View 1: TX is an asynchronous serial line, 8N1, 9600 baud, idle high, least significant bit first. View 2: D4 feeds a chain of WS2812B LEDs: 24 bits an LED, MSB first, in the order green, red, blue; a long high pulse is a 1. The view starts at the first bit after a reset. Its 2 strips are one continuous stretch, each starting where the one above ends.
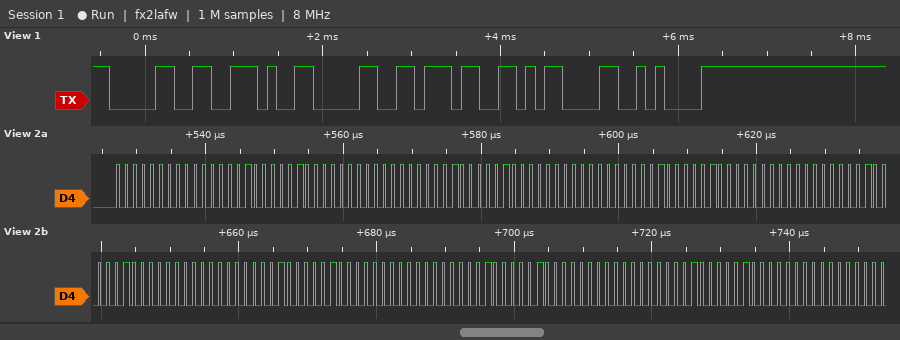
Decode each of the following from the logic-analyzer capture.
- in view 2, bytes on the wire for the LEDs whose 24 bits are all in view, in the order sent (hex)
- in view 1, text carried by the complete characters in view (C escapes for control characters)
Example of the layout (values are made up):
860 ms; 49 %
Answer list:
00 01 04 00 01 04 00 01 04 00 01 04 00 01 04 00 01 04 00 01 04; "0.07\r\n"
